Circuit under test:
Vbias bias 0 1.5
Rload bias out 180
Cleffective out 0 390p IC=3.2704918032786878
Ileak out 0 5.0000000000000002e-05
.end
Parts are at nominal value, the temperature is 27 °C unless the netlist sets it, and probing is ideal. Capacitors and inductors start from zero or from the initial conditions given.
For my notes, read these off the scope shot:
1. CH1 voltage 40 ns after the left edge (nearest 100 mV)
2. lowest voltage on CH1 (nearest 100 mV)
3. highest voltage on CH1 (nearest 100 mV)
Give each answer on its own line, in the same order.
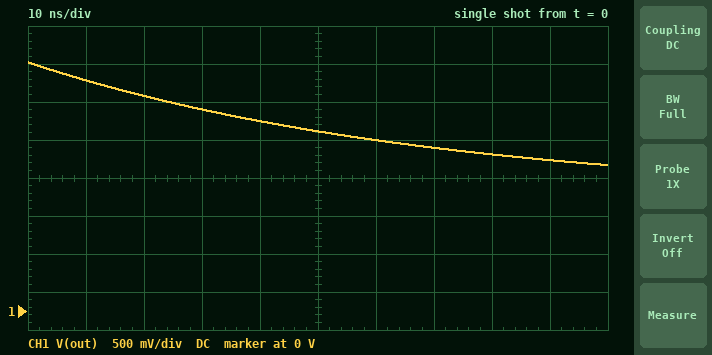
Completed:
2.5 V
1.9 V
3.3 V
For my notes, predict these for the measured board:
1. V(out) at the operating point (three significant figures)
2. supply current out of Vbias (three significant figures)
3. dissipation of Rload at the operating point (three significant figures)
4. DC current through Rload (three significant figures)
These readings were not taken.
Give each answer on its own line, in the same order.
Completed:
1.49 V
50.0 µA
450 nW
50.0 µA
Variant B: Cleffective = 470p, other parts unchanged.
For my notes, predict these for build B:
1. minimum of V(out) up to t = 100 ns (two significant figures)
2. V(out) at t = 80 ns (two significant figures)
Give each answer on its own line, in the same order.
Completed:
2.0 V
2.2 V
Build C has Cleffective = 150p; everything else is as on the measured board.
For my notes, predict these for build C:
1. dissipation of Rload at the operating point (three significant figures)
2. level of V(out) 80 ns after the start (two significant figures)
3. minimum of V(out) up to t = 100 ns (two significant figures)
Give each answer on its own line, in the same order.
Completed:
450 nW
1.6 V
1.5 V
